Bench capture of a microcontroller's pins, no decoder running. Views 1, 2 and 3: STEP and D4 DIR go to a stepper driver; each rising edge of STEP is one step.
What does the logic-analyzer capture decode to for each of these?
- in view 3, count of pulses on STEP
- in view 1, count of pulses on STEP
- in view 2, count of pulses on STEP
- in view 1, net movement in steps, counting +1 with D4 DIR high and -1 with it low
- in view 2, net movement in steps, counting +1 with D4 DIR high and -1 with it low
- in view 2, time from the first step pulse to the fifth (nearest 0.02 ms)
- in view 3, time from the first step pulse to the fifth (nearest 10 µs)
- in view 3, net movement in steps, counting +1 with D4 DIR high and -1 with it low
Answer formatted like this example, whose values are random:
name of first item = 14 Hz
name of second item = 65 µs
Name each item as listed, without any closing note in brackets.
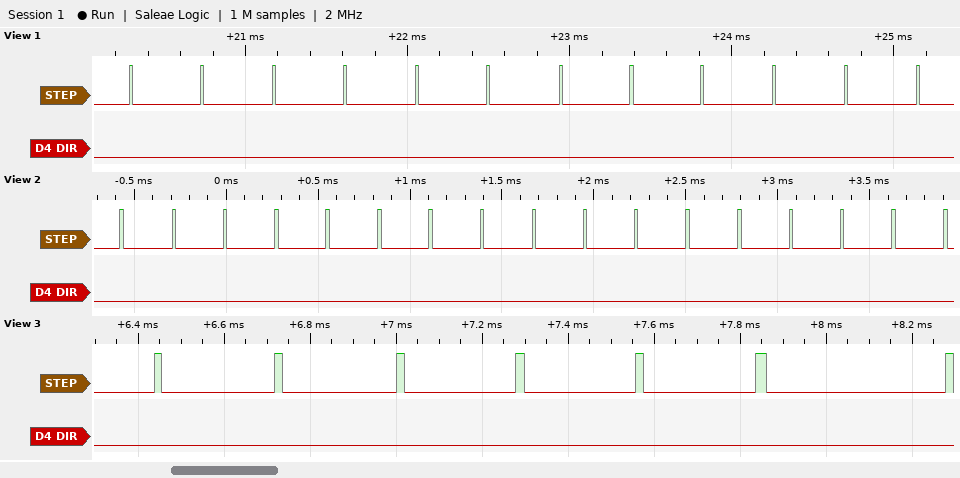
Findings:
in view 3, count of pulses on STEP = 7
in view 1, count of pulses on STEP = 12
in view 2, count of pulses on STEP = 17
in view 1, net movement in steps, counting +1 with D4 DIR high and -1 with it low = -12
in view 2, net movement in steps, counting +1 with D4 DIR high and -1 with it low = -17
in view 2, time from the first step pulse to the fifth = 1.12 ms
in view 3, time from the first step pulse to the fifth = 1120 µs
in view 3, net movement in steps, counting +1 with D4 DIR high and -1 with it low = -7
